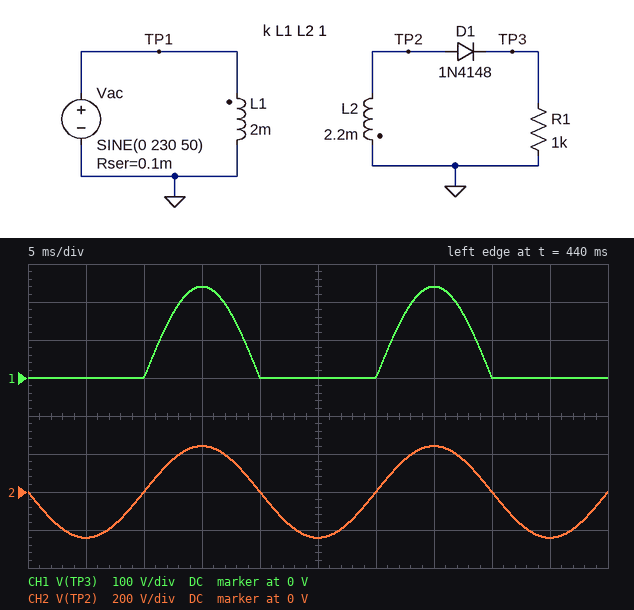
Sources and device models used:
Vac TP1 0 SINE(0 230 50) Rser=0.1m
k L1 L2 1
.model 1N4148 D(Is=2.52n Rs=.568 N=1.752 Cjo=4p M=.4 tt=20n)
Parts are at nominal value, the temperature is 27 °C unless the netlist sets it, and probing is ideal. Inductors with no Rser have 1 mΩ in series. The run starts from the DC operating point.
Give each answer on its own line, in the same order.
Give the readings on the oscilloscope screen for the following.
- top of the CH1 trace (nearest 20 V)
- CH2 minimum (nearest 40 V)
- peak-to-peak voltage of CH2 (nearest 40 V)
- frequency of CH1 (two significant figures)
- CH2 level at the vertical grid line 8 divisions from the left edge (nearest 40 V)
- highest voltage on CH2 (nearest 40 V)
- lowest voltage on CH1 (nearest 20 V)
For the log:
240 V
-240 V
480 V
50 Hz
0 V
240 V
0 V
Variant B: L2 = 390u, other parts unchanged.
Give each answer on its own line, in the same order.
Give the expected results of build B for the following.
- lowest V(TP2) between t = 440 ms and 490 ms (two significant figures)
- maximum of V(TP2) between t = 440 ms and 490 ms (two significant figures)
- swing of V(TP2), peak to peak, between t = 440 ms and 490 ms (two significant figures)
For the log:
-100 V
100 V
200 V
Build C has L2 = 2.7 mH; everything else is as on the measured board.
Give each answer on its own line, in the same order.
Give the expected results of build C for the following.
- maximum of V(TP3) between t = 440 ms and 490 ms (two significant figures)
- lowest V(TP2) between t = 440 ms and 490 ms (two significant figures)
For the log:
270 V
-270 V
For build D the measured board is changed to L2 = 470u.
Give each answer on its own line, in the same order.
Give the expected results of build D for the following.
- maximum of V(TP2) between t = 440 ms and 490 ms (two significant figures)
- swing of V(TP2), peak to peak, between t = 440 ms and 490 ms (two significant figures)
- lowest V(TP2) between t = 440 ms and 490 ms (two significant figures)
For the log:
110 V
220 V
-110 V
